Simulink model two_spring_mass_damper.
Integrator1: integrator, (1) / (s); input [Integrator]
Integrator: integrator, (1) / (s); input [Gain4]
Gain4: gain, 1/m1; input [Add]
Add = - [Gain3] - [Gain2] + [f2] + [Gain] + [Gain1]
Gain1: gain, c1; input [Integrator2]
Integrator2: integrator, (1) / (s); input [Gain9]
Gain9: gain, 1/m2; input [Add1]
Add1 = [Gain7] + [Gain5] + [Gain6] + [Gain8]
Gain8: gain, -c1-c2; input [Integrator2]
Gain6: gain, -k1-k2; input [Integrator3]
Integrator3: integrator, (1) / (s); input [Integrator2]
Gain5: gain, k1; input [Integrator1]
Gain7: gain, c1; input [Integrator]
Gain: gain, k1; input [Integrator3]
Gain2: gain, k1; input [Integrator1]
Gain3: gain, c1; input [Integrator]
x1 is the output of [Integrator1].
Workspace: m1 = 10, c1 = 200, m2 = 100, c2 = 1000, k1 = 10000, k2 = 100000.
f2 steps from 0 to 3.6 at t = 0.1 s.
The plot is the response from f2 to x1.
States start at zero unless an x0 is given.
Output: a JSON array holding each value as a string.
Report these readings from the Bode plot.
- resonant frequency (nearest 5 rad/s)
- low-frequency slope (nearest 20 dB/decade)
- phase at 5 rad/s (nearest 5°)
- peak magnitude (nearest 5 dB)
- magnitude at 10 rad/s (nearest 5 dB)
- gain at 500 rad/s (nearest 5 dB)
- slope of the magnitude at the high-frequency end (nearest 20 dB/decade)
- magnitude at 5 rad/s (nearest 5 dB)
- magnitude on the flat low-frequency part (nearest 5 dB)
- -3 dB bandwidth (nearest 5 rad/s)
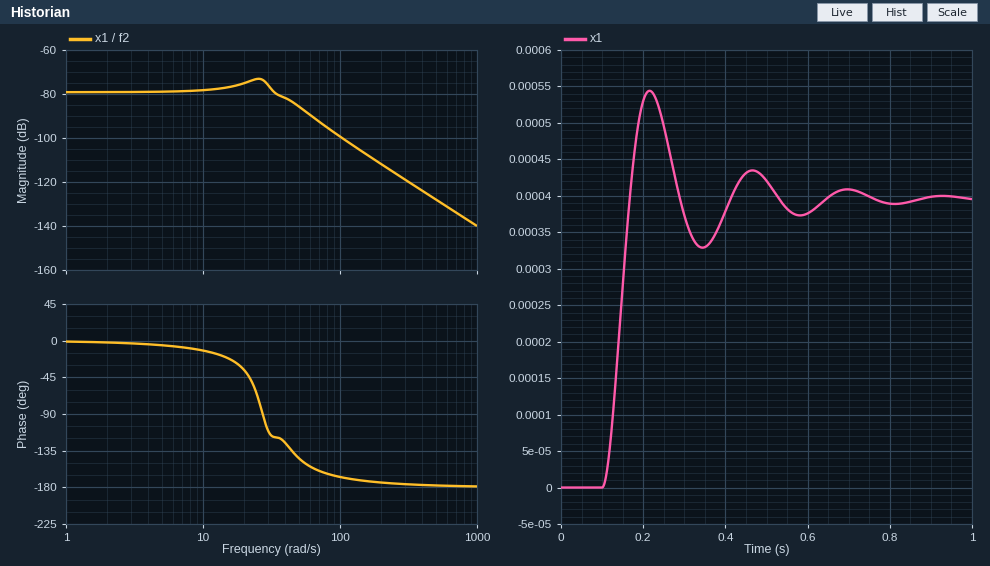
["25 rad/s", "0 dB/decade", "-5°", "-75 dB", "-80 dB", "-130 dB", "-40 dB/decade", "-80 dB", "-80 dB", "40 rad/s"]
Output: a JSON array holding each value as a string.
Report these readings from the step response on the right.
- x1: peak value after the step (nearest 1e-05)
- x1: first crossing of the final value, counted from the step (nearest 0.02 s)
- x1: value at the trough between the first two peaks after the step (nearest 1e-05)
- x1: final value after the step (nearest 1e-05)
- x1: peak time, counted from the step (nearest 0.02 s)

["0.00054", "0.06 s", "0.00033", "0.00040", "0.12 s"]
